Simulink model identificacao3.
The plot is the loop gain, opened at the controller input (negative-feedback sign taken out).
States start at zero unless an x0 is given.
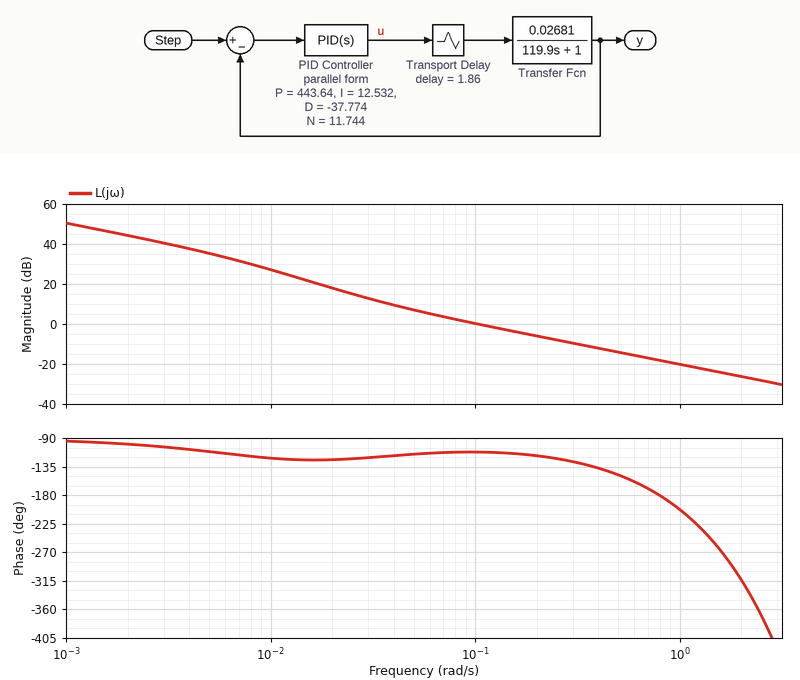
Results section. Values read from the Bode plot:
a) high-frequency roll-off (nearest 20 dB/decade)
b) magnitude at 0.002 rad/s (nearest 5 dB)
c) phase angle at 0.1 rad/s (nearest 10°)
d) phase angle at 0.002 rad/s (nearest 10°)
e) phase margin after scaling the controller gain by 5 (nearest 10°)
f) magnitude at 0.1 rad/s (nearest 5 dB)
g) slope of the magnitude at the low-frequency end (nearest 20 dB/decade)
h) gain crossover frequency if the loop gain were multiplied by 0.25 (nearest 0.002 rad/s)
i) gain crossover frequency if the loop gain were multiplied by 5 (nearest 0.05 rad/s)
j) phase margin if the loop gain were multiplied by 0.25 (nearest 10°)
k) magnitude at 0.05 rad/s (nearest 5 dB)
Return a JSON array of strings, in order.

["-20 dB/decade", "45 dB", "-110°", "-100°", "30°", "0 dB", "-20 dB/decade", "0.032 rad/s", "0.50 rad/s", "60°", "5 dB"]
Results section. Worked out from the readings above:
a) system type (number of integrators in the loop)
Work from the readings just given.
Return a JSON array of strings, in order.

["1"]
